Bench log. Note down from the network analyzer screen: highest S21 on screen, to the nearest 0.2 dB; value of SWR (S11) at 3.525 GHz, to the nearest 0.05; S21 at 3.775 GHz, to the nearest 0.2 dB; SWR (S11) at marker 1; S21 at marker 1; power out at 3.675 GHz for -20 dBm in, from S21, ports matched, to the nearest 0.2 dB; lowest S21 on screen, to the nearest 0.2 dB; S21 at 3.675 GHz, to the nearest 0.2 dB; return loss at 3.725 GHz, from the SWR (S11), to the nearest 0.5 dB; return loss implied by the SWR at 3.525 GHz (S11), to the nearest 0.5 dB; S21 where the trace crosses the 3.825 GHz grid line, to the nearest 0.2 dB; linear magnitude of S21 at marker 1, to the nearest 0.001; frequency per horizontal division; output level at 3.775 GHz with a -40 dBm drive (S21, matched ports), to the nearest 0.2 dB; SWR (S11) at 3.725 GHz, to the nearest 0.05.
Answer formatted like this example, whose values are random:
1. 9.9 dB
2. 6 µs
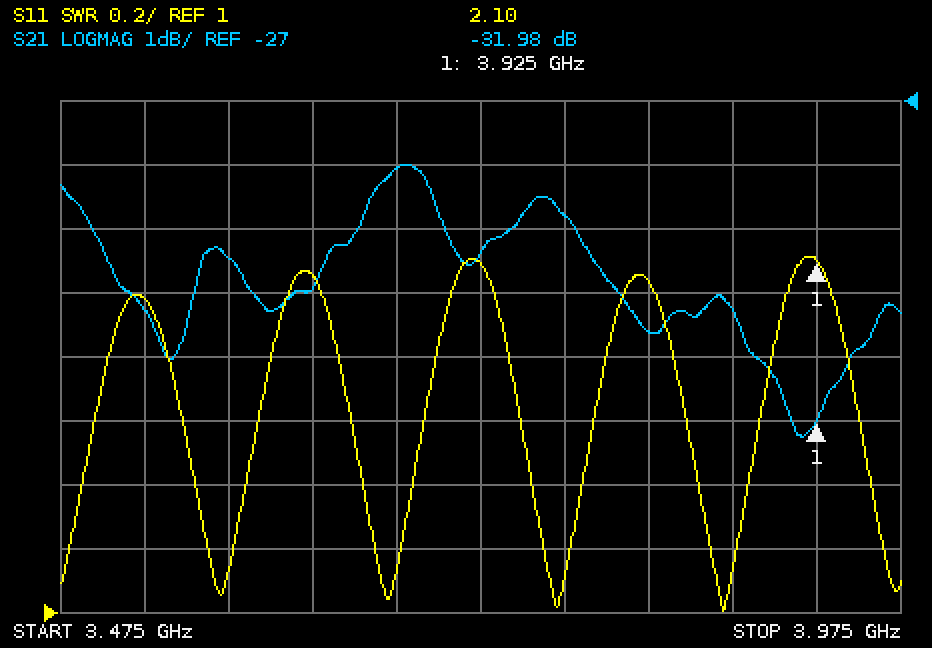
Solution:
1. -28.0 dB
2. 2.00
3. -28.8 dB
4. 2.10
5. -31.98 dB
6. -48.0 dBm
7. -32.2 dB
8. -28.0 dB
9. 9.0 dB
10. 9.5 dB
11. -30.6 dB
12. 0.025
13. 50 MHz
14. -68.8 dBm
15. 2.10
